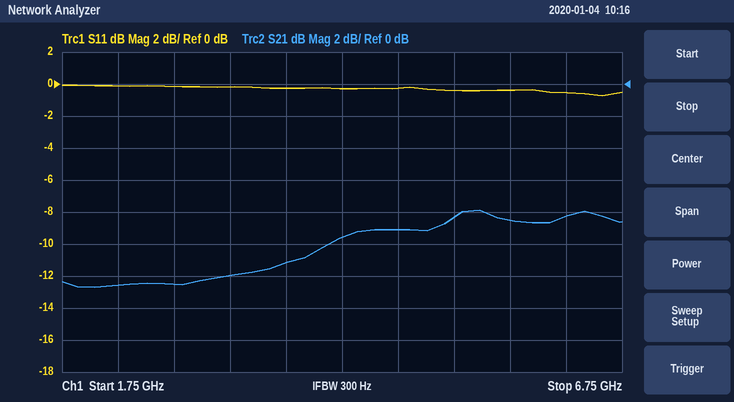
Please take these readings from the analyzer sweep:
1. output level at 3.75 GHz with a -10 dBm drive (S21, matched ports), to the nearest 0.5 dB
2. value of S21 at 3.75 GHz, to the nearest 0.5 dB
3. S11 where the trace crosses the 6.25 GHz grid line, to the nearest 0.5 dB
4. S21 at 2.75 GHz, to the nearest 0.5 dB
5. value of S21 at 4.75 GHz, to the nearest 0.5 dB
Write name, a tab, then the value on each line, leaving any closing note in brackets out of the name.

output level at 3.75 GHz with a -10 dBm drive (S21, matched ports), to the nearest 0.5 dB	-21.0 dBm
value of S21 at 3.75 GHz, to the nearest 0.5 dB	-11.0 dB
S11 where the trace crosses the 6.25 GHz grid line, to the nearest 0.5 dB	-0.5 dB
S21 at 2.75 GHz, to the nearest 0.5 dB	-12.5 dB
value of S21 at 4.75 GHz, to the nearest 0.5 dB	-9.0 dB
